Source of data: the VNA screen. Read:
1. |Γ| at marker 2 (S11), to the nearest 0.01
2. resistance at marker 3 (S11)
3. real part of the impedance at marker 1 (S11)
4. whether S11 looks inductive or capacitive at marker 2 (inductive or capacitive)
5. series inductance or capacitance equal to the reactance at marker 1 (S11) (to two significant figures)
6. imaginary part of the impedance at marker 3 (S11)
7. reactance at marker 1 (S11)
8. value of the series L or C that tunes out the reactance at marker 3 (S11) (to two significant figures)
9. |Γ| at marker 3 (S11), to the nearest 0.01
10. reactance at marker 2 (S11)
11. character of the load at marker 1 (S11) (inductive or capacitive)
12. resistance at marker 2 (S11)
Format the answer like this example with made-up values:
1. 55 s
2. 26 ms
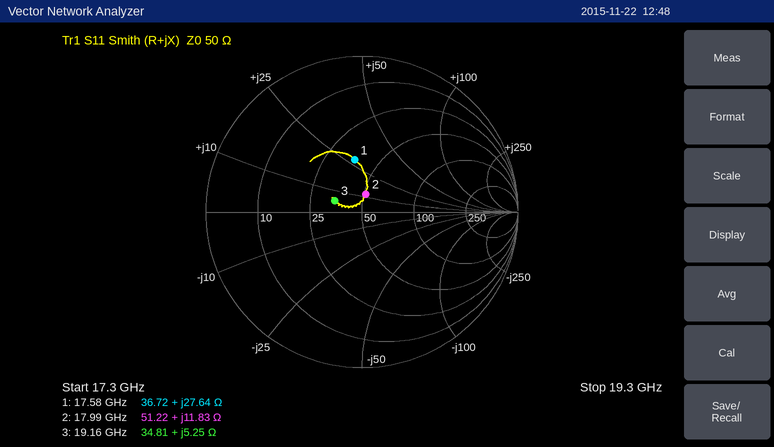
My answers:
1. 0.12
2. 34.81 Ω
3. 36.72 Ω
4. inductive
5. 250 pH
6. +5.25 Ω
7. +27.64 Ω
8. 1.6 pF
9. 0.19
10. +11.83 Ω
11. inductive
12. 51.22 Ω
